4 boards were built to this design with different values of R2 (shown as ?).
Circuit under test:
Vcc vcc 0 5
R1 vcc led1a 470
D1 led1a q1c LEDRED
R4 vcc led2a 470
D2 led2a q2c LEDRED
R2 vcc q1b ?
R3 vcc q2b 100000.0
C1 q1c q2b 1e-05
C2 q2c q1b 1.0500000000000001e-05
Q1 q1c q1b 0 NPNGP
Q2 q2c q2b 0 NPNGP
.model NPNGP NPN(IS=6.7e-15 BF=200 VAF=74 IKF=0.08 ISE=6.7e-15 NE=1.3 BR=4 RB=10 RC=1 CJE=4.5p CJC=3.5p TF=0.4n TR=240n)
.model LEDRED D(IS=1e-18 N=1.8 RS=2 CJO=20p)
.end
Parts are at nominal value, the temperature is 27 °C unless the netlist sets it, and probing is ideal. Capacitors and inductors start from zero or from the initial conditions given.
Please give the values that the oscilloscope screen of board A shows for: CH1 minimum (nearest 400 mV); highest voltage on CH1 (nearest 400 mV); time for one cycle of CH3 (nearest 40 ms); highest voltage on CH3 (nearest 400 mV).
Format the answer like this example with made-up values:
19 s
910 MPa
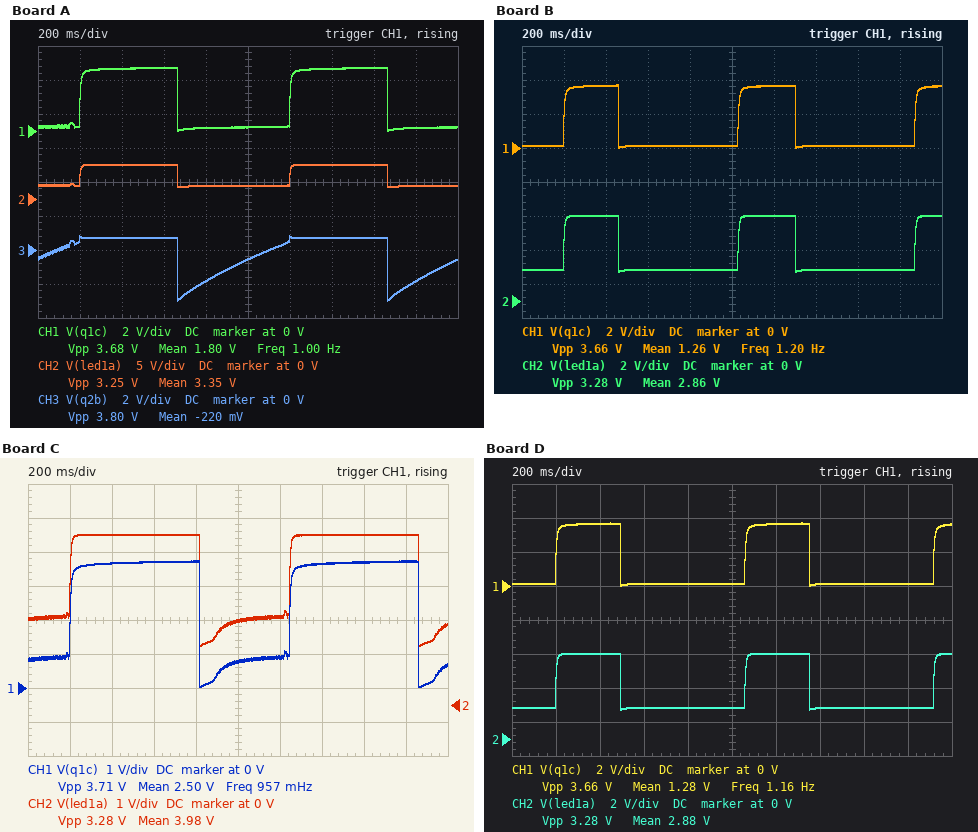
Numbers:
0 V
3.6 V
1.00 s
800 mV
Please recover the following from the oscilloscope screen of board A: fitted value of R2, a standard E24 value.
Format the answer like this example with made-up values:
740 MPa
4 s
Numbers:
91 kΩ
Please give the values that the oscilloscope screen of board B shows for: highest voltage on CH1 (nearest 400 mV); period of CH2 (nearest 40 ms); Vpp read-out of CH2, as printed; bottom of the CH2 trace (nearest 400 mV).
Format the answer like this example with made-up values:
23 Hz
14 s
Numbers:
3.6 V
840 ms
3.28 V
1.6 V
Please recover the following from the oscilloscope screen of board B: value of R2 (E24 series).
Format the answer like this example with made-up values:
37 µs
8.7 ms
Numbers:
51 kΩ
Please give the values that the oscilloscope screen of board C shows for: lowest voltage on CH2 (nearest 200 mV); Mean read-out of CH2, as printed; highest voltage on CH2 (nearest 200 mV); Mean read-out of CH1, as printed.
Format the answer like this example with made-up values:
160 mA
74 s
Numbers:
1.8 V
3.98 V
5.0 V
2.50 V
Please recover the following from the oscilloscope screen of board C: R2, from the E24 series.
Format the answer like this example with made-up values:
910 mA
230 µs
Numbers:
120 kΩ
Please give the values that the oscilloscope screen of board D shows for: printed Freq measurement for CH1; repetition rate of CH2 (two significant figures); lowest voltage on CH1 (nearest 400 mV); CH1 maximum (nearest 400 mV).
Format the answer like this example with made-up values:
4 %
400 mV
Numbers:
1.16 Hz
1.2 Hz
0 V
3.6 V
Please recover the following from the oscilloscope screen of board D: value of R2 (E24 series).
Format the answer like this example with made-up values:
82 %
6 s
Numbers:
56 kΩ
